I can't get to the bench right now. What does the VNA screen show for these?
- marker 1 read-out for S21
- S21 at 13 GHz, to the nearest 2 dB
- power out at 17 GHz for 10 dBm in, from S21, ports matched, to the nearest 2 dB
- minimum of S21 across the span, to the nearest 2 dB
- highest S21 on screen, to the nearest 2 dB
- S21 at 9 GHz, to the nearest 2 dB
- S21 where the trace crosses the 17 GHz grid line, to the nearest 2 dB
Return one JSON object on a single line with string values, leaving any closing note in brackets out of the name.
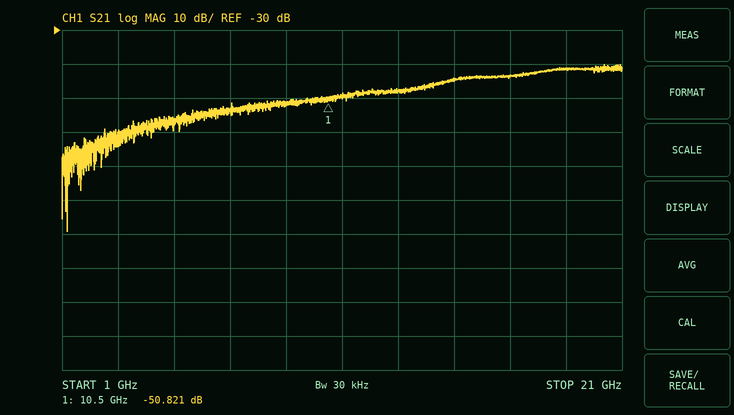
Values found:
{"marker 1 read-out for S21": "-50.821 dB", "S21 at 13 GHz, to the nearest 2 dB": "-48 dB", "power out at 17 GHz for 10 dBm in, from S21, ports matched, to the nearest 2 dB": "-34 dBm", "minimum of S21 across the span, to the nearest 2 dB": "-90 dB", "highest S21 on screen, to the nearest 2 dB": "-40 dB", "S21 at 9 GHz, to the nearest 2 dB": "-52 dB", "S21 where the trace crosses the 17 GHz grid line, to the nearest 2 dB": "-44 dB"}
